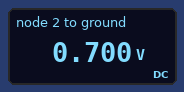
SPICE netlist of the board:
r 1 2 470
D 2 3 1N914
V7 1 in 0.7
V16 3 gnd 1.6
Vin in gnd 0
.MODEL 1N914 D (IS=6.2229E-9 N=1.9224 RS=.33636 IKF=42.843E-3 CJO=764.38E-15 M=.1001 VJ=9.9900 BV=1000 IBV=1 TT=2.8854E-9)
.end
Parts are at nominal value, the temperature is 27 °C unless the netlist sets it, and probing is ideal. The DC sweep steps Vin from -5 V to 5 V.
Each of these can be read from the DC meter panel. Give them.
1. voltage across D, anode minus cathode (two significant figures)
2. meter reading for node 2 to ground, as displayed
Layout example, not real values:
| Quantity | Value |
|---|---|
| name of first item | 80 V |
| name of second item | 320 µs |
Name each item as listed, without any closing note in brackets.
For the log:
| Quantity | Value |
|---|---|
| voltage across D, anode minus cathode | -900 mV |
| meter reading for node 2 to ground, as displayed | 0.700 V |
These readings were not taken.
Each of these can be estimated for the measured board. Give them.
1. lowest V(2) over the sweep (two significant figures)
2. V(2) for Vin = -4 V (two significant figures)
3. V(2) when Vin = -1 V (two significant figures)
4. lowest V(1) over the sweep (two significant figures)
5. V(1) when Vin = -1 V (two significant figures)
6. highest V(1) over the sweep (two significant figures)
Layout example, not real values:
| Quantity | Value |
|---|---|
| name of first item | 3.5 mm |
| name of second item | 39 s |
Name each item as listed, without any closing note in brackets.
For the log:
| Quantity | Value |
|---|---|
| lowest V(2) over the sweep | -4.3 V |
| V(2) for Vin = -4 V | -3.3 V |
| V(2) when Vin = -1 V | -300 mV |
| lowest V(1) over the sweep | -4.3 V |
| V(1) when Vin = -1 V | -300 mV |
| highest V(1) over the sweep | 5.7 V |
